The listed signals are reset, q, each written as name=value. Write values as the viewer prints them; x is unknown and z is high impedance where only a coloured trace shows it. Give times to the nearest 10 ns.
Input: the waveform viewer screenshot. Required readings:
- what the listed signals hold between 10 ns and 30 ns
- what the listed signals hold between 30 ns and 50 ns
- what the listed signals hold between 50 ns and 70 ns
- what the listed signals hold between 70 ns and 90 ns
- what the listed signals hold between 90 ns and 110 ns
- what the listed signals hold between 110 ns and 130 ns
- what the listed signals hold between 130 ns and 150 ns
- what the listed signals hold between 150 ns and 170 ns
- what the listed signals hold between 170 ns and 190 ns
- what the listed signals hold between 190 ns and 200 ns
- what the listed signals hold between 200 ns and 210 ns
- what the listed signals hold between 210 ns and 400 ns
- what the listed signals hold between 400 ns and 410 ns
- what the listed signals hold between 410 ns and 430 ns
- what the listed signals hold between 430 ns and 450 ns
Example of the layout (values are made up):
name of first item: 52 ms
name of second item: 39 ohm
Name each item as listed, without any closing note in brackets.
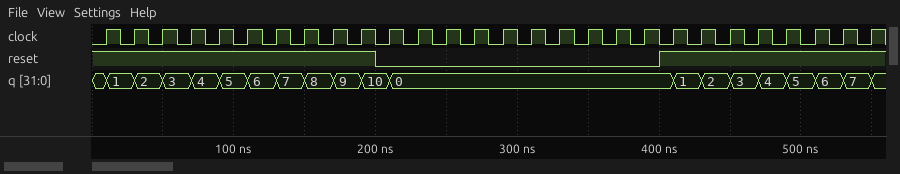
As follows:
what the listed signals hold between 10 ns and 30 ns: reset=1, q=1
what the listed signals hold between 30 ns and 50 ns: reset=1, q=2
what the listed signals hold between 50 ns and 70 ns: reset=1, q=3
what the listed signals hold between 70 ns and 90 ns: reset=1, q=4
what the listed signals hold between 90 ns and 110 ns: reset=1, q=5
what the listed signals hold between 110 ns and 130 ns: reset=1, q=6
what the listed signals hold between 130 ns and 150 ns: reset=1, q=7
what the listed signals hold between 150 ns and 170 ns: reset=1, q=8
what the listed signals hold between 170 ns and 190 ns: reset=1, q=9
what the listed signals hold between 190 ns and 200 ns: reset=1, q=10
what the listed signals hold between 200 ns and 210 ns: reset=0, q=10
what the listed signals hold between 210 ns and 400 ns: reset=0, q=0
what the listed signals hold between 400 ns and 410 ns: reset=1, q=0
what the listed signals hold between 410 ns and 430 ns: reset=1, q=1
what the listed signals hold between 430 ns and 450 ns: reset=1, q=2
